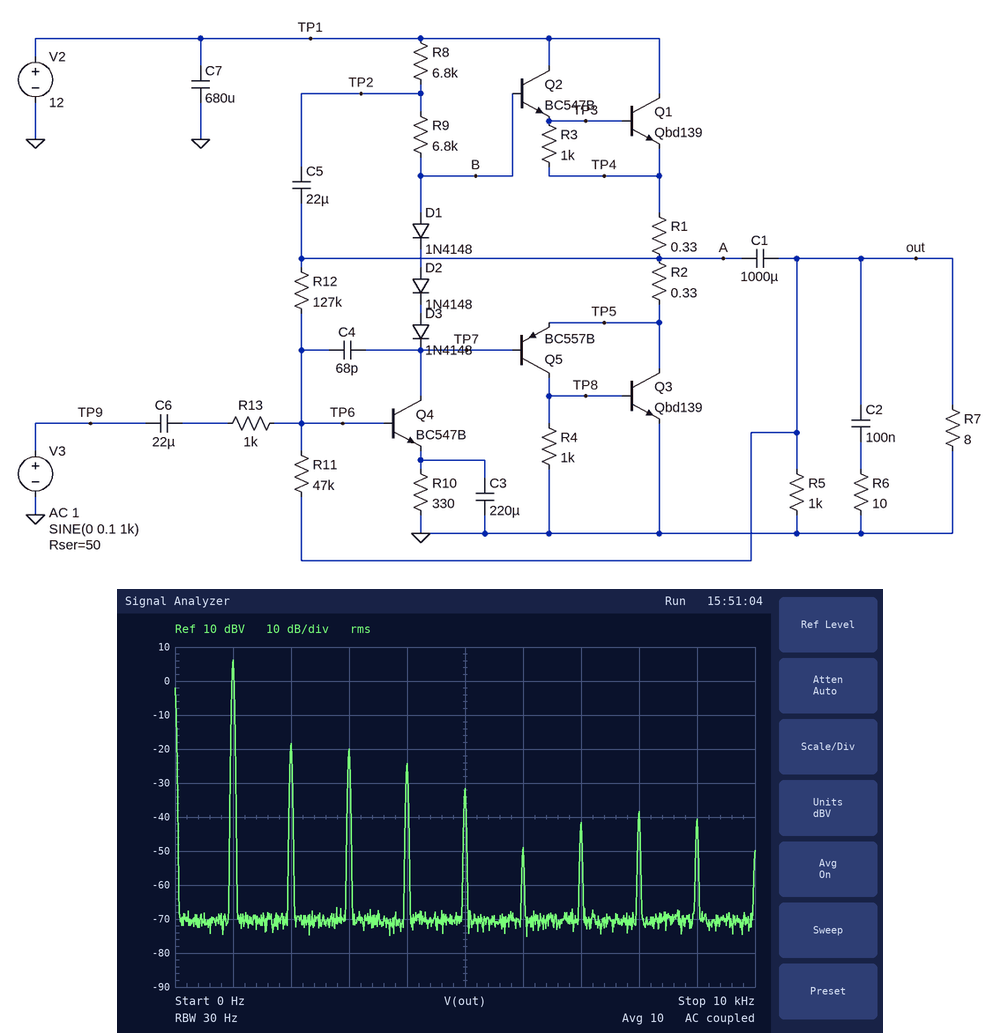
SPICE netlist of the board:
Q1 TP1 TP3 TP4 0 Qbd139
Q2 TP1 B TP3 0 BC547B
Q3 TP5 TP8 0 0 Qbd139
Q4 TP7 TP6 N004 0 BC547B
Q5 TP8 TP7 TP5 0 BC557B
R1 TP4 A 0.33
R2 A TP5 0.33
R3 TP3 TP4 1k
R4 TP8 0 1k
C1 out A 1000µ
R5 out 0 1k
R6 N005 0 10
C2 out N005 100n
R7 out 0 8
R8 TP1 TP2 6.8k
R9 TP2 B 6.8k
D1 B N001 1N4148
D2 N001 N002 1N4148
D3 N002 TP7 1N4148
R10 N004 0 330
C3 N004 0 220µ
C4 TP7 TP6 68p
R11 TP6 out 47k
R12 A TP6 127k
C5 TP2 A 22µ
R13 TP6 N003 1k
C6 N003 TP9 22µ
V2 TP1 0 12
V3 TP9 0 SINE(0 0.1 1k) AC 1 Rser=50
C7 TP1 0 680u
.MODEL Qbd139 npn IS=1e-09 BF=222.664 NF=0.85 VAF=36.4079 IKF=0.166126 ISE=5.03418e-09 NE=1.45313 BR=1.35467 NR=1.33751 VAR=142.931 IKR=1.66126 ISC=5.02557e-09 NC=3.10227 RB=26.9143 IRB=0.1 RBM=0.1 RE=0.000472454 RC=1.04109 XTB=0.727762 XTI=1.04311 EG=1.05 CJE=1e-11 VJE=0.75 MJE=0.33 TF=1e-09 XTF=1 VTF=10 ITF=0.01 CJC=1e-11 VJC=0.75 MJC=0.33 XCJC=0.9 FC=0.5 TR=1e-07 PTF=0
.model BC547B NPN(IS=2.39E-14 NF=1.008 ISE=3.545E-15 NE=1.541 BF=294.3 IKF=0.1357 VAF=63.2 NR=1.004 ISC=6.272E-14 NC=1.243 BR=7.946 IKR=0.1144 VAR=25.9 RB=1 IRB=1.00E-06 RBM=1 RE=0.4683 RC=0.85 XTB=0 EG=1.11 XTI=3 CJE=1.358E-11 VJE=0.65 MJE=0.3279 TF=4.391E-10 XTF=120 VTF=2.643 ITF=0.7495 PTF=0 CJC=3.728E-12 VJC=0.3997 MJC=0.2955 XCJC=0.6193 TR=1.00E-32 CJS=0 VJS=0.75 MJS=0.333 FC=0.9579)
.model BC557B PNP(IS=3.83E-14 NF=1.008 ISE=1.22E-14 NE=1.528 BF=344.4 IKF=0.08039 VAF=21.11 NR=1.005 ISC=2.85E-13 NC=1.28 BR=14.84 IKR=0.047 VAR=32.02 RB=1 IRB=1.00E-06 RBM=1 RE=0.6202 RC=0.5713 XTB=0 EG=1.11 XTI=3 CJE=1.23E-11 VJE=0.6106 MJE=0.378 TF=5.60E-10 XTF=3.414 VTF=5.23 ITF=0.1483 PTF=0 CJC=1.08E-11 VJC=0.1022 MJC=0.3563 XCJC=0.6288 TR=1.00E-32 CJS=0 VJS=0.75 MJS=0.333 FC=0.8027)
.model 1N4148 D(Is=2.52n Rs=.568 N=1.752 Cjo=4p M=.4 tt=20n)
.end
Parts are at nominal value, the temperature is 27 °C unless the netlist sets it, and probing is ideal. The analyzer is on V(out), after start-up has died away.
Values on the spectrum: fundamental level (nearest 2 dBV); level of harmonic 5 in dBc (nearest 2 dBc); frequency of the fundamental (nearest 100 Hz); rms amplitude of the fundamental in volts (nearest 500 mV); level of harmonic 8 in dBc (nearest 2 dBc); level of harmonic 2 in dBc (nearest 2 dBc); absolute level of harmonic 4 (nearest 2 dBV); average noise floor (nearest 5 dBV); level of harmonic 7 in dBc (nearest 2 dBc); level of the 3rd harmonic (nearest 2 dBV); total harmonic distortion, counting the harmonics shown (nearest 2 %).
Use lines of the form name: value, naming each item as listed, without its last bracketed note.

fundamental level: 6 dBV
level of harmonic 5 in dBc: -38 dBc
frequency of the fundamental: 1.0 kHz
rms amplitude of the fundamental in volts: 2.0 V
level of harmonic 8 in dBc: -44 dBc
level of harmonic 2 in dBc: -24 dBc
absolute level of harmonic 4: -24 dBV
average noise floor: -70 dBV
level of harmonic 7 in dBc: -48 dBc
level of the 3rd harmonic: -20 dBV
total harmonic distortion, counting the harmonics shown: 8 %
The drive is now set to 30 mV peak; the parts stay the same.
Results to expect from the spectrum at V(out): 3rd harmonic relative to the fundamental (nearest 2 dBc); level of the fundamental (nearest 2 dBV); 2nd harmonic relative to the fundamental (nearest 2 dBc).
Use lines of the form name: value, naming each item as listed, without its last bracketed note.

3rd harmonic relative to the fundamental: -56 dBc
level of the fundamental: -4 dBV
2nd harmonic relative to the fundamental: -52 dBc
